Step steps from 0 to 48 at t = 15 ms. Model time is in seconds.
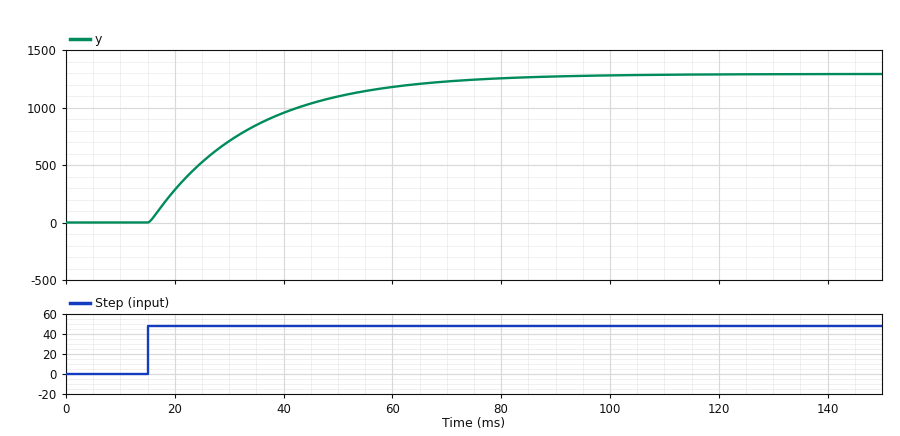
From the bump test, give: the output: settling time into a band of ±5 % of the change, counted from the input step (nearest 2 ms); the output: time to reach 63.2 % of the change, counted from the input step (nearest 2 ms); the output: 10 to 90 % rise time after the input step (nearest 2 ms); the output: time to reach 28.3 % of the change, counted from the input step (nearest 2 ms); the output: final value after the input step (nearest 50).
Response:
56 ms
18 ms
40 ms
6 ms
1300
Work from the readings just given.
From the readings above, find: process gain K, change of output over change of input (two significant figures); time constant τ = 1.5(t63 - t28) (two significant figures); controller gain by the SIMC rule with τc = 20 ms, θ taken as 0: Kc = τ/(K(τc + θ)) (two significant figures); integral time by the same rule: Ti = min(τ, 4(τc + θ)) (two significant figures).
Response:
27
18 ms
0.033
18 ms
